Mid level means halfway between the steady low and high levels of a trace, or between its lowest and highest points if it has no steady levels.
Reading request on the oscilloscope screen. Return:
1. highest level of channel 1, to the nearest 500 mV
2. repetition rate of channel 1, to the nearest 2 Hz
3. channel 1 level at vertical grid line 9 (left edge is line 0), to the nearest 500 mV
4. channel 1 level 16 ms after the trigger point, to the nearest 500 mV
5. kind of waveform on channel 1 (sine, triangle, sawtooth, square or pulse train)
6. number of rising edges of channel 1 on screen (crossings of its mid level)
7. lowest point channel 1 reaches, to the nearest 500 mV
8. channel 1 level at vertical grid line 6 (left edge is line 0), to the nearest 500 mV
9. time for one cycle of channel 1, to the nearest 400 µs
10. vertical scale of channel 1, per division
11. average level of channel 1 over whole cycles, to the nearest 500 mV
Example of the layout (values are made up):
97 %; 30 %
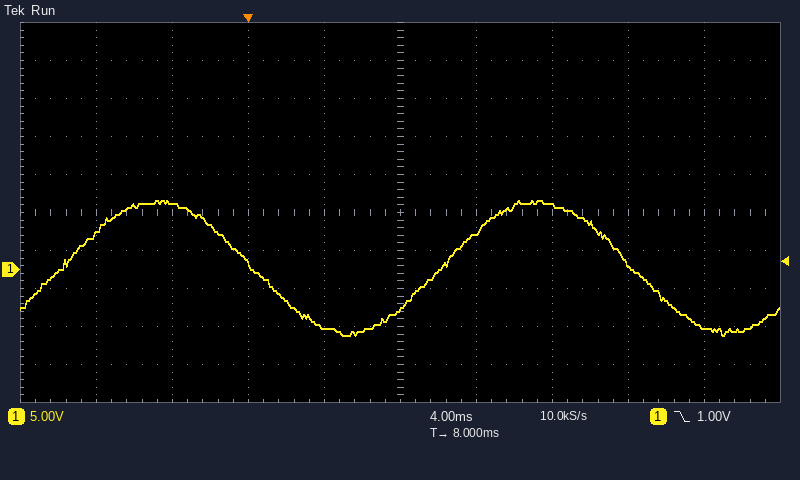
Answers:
9.0 V; 50 Hz; -7.5 V; 8.5 V; sine; 2; -8.5 V; 5.0 V; 20.0 ms; 5 V; 500 mV
